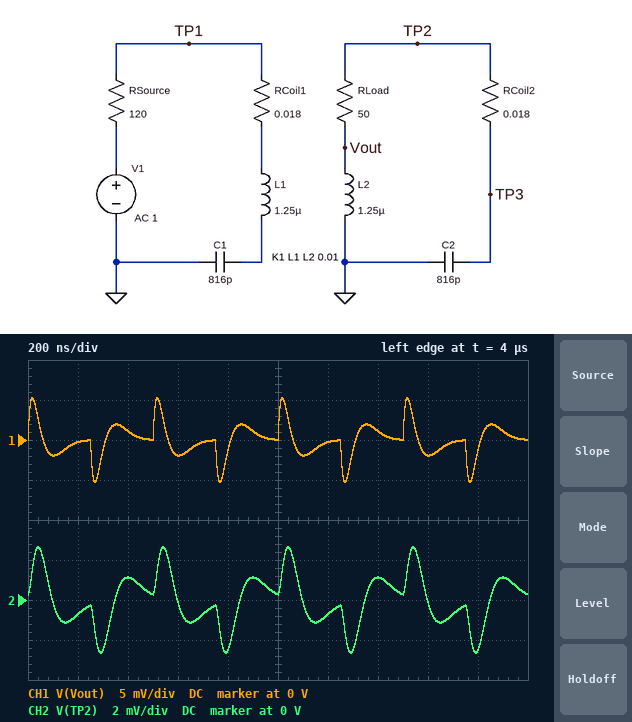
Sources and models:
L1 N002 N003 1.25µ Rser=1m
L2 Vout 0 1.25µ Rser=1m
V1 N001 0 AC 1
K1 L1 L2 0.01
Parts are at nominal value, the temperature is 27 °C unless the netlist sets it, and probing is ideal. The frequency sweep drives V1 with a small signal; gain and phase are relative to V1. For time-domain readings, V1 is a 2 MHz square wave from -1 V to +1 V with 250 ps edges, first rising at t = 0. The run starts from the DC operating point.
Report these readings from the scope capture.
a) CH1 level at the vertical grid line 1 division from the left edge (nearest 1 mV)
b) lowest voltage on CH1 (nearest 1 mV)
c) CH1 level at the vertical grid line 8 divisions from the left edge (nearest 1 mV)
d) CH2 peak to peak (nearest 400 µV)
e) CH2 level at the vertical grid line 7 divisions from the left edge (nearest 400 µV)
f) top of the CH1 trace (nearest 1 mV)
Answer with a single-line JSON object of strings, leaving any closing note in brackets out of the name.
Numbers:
{"CH1 level at the vertical grid line 1 division from the left edge": "0 V", "lowest voltage on CH1": "-5 mV", "CH1 level at the vertical grid line 8 divisions from the left edge": "-2 mV", "CH2 peak to peak": "5.2 mV", "CH2 level at the vertical grid line 7 divisions from the left edge": "1.2 mV", "top of the CH1 trace": "5 mV"}
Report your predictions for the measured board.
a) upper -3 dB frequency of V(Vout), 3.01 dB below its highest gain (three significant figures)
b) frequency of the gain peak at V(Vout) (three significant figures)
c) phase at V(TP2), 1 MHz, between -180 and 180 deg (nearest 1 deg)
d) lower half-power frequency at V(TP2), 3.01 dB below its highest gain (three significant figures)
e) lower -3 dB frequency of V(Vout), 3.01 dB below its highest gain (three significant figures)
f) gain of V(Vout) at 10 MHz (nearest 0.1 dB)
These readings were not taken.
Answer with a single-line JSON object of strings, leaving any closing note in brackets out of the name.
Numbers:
{"upper -3 dB frequency of V(Vout), 3.01 dB below its highest gain": "15.8 MHz", "frequency of the gain peak at V(Vout)": "6.66 MHz", "phase at V(TP2), 1 MHz, between -180 and 180 deg": "132 deg", "lower half-power frequency at V(TP2), 3.01 dB below its highest gain": "2.92 MHz", "lower -3 dB frequency of V(Vout), 3.01 dB below its highest gain": "3.76 MHz", "gain of V(Vout) at 10 MHz": "-47.8 dB"}
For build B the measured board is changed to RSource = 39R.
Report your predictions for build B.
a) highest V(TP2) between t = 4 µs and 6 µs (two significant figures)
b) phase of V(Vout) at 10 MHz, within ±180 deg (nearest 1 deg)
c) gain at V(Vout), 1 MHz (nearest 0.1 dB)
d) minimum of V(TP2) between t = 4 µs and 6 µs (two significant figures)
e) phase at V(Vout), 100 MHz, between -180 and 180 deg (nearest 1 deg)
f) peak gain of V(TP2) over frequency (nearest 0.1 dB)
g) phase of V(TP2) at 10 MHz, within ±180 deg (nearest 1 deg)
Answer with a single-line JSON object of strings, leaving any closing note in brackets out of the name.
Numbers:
{"highest V(TP2) between t = 4 µs and 6 µs": "4.5 mV", "phase of V(Vout) at 10 MHz, within ±180 deg": "-38 deg", "gain at V(Vout), 1 MHz": "-67.4 dB", "minimum of V(TP2) between t = 4 µs and 6 µs": "-4.5 mV", "phase at V(Vout), 100 MHz, between -180 and 180 deg": "-86 deg", "peak gain of V(TP2) over frequency": "-42.1 dB", "phase of V(TP2) at 10 MHz, within ±180 deg": "-106 deg"}
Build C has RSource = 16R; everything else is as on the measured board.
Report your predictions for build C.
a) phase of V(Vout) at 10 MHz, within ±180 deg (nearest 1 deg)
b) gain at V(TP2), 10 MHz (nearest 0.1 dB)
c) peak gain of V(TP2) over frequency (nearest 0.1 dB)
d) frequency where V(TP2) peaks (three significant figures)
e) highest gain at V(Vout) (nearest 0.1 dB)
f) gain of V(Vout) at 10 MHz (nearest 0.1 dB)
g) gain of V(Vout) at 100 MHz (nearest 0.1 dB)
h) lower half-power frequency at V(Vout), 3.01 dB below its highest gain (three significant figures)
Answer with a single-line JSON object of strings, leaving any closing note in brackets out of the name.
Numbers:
{"phase of V(Vout) at 10 MHz, within ±180 deg": "-56 deg", "gain at V(TP2), 10 MHz": "-49.8 dB", "peak gain of V(TP2) over frequency": "-34.4 dB", "frequency where V(TP2) peaks": "4.98 MHz", "highest gain at V(Vout)": "-30.1 dB", "gain of V(Vout) at 10 MHz": "-41.0 dB", "gain of V(Vout) at 100 MHz": "-63.9 dB", "lower half-power frequency at V(Vout), 3.01 dB below its highest gain": "4.28 MHz"}
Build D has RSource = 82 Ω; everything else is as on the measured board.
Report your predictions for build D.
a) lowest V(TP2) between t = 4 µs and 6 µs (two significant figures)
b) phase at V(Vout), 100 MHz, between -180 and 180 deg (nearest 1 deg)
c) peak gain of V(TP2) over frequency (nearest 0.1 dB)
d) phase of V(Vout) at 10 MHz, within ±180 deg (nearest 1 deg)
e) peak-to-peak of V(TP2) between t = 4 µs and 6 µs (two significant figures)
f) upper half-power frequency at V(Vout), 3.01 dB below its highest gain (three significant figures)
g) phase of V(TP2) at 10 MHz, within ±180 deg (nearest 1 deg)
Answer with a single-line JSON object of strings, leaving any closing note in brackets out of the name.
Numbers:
{"lowest V(TP2) between t = 4 µs and 6 µs": "-3.3 mV", "phase at V(Vout), 100 MHz, between -180 and 180 deg": "-83 deg", "peak gain of V(TP2) over frequency": "-48.6 dB", "phase of V(Vout) at 10 MHz, within ±180 deg": "-17 deg", "peak-to-peak of V(TP2) between t = 4 µs and 6 µs": "6.6 mV", "upper half-power frequency at V(Vout), 3.01 dB below its highest gain": "12.5 MHz", "phase of V(TP2) at 10 MHz, within ±180 deg": "-85 deg"}
